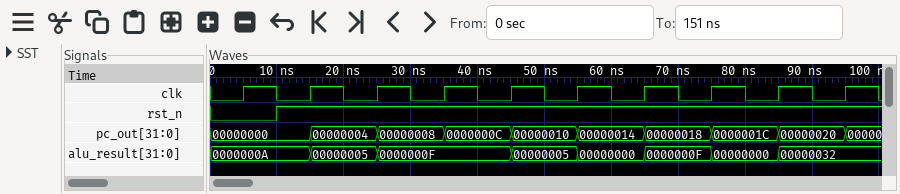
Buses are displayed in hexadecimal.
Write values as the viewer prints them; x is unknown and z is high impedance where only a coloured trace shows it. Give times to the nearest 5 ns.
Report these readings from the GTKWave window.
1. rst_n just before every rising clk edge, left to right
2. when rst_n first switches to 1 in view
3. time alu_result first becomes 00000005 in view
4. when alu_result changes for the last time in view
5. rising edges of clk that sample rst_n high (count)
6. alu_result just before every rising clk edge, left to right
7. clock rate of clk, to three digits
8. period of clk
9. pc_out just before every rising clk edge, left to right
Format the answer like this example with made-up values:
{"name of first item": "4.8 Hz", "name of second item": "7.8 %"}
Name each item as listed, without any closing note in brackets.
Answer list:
{"rst_n just before every rising clk edge, left to right": "0 1 1 1 1 1 1 1 1 1", "when rst_n first switches to 1 in view": "10 ns", "time alu_result first becomes 00000005 in view": "15 ns", "when alu_result changes for the last time in view": "85 ns", "rising edges of clk that sample rst_n high": "9", "alu_result just before every rising clk edge, left to right": "0000000A, 0000000A, 00000005, 0000000F, 0000000F, 00000005, 00000000, 0000000F, 00000000, 00000032", "clock rate of clk, to three digits": "100 MHz", "period of clk": "10 ns", "pc_out just before every rising clk edge, left to right": "00000000, 00000000, 00000004, 00000008, 0000000C, 00000010, 00000014, 00000018, 0000001C, 00000020"}
